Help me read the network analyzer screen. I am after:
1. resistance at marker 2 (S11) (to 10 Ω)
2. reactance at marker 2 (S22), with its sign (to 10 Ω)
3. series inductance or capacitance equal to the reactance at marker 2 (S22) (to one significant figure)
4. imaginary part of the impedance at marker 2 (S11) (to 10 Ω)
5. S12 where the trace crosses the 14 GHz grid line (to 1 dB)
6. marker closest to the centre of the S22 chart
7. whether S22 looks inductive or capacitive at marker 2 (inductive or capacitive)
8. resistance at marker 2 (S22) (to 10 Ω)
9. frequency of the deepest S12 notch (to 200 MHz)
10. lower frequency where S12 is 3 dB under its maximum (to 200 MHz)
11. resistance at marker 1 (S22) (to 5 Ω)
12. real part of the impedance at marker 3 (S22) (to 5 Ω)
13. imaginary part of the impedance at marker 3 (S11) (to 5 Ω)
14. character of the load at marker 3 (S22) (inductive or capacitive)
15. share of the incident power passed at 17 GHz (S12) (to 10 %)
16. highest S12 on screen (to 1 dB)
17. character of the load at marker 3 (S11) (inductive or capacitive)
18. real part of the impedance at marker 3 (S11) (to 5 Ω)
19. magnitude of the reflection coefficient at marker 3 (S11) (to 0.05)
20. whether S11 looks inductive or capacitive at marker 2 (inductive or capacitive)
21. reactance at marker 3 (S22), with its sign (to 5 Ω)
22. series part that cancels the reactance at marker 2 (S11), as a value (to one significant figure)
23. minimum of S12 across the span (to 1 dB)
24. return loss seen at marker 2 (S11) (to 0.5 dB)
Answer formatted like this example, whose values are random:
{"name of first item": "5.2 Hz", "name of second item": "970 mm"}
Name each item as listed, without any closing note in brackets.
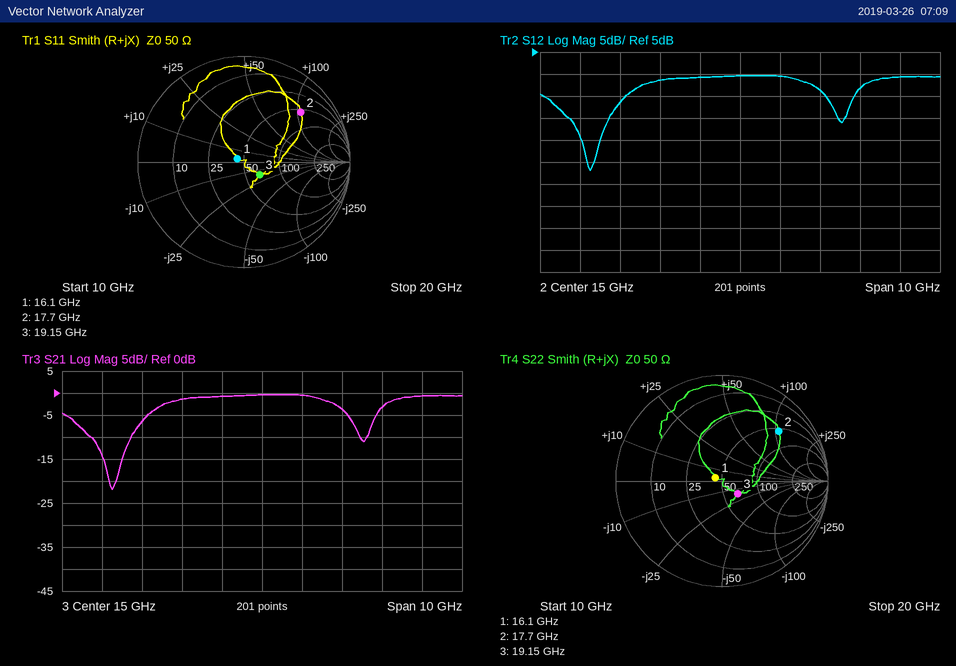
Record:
{"resistance at marker 2 (S11)": "60 Ω", "reactance at marker 2 (S22), with its sign": "+110 Ω", "series inductance or capacitance equal to the reactance at marker 2 (S22)": "1.0 nH", "imaginary part of the impedance at marker 2 (S11)": "+110 Ω", "S12 where the trace crosses the 14 GHz grid line": "-1 dB", "marker closest to the centre of the S22 chart": "marker 1", "whether S22 looks inductive or capacitive at marker 2": "inductive", "resistance at marker 2 (S22)": "60 Ω", "frequency of the deepest S12 notch": "11.2 GHz", "lower frequency where S12 is 3 dB under its maximum": "12.4 GHz", "resistance at marker 1 (S22)": "45 Ω", "real part of the impedance at marker 3 (S22)": "65 Ω", "imaginary part of the impedance at marker 3 (S11)": "-15 Ω", "character of the load at marker 3 (S22)": "capacitive", "share of the incident power passed at 17 GHz (S12)": "40 %", "highest S12 on screen": "0 dB", "character of the load at marker 3 (S11)": "capacitive", "real part of the impedance at marker 3 (S11)": "65 Ω", "magnitude of the reflection coefficient at marker 3 (S11)": "0.20", "whether S11 looks inductive or capacitive at marker 2": "inductive", "reactance at marker 3 (S22), with its sign": "-15 Ω", "series part that cancels the reactance at marker 2 (S11), as a value": "80 fF", "minimum of S12 across the span": "-22 dB", "return loss seen at marker 2 (S11)": "3.0 dB"}
